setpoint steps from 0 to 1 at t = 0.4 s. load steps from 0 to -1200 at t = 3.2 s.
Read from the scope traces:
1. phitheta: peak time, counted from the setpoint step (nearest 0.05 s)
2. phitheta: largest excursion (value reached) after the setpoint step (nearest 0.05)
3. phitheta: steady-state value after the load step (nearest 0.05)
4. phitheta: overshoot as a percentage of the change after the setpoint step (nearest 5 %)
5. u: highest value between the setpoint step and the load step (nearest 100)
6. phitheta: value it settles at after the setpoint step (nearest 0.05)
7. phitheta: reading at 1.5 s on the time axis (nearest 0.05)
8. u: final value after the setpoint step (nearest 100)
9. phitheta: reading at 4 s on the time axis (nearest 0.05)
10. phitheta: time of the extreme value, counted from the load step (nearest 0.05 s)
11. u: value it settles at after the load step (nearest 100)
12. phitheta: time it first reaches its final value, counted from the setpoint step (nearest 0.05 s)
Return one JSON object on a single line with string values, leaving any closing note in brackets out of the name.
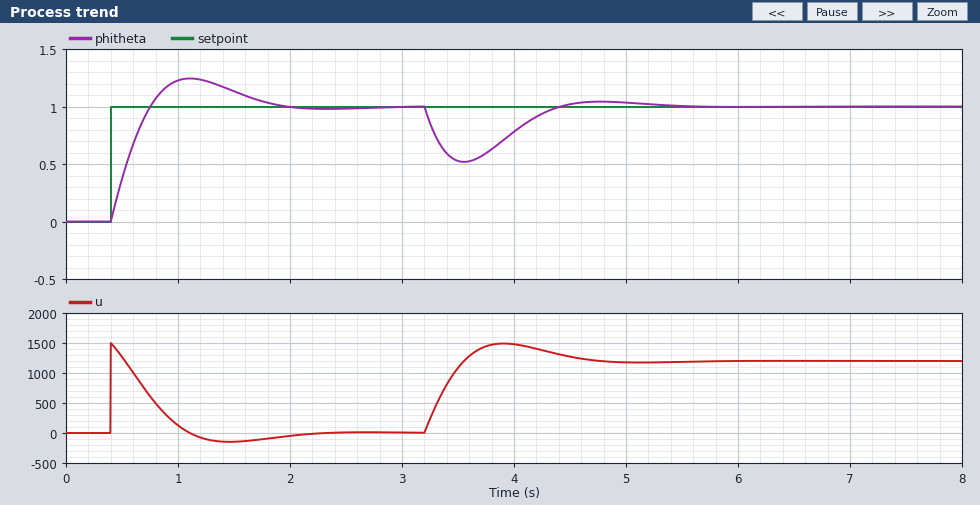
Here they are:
{"phitheta: peak time, counted from the setpoint step": "0.70 s", "phitheta: largest excursion (value reached) after the setpoint step": "1.25", "phitheta: steady-state value after the load step": "1.00", "phitheta: overshoot as a percentage of the change after the setpoint step": "25 %", "u: highest value between the setpoint step and the load step": "1500", "phitheta: value it settles at after the setpoint step": "1.00", "phitheta: reading at 1.5 s on the time axis": "1.15", "u: final value after the setpoint step": "0", "phitheta: reading at 4 s on the time axis": "0.80", "phitheta: time of the extreme value, counted from the load step": "0.35 s", "u: value it settles at after the load step": "1200", "phitheta: time it first reaches its final value, counted from the setpoint step": "0.35 s"}
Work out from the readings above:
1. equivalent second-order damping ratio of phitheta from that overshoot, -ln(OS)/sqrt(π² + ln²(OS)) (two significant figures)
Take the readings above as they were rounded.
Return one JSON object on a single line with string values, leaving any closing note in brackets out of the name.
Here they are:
{"equivalent second-order damping ratio of phitheta from that overshoot, -ln(OS)/sqrt(π² + ln²(OS))": "0.40"}
